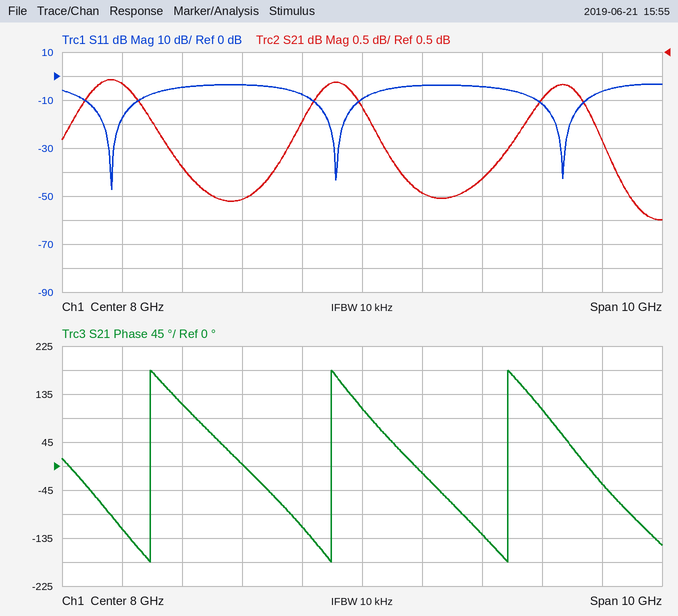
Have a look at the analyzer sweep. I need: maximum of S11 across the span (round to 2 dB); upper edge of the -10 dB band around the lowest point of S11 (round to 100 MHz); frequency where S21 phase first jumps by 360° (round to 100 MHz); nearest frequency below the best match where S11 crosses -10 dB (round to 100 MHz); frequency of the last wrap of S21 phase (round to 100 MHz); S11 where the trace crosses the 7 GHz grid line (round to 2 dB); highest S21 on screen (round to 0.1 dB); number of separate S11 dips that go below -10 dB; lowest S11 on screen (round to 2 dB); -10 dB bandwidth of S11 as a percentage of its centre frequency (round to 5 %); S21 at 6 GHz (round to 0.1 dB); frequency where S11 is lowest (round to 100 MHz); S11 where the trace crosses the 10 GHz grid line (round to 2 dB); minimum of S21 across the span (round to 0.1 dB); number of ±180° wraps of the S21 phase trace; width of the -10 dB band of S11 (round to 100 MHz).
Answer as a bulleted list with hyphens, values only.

- -4 dB
- 4.3 GHz
- 4.5 GHz
- 3.4 GHz
- 10.4 GHz
- -8 dB
- -0.1 dB
- 3
- -48 dB
- 25 %
- -2.6 dB
- 3.8 GHz
- -4 dB
- -3.0 dB
- 3
- 900 MHz
